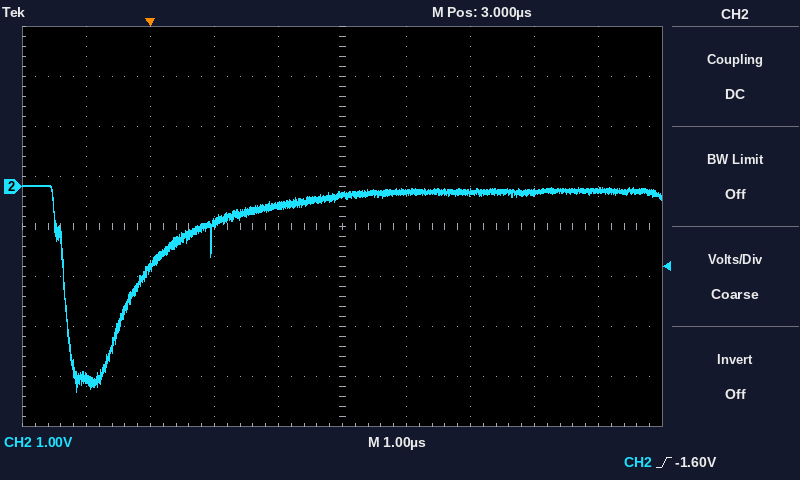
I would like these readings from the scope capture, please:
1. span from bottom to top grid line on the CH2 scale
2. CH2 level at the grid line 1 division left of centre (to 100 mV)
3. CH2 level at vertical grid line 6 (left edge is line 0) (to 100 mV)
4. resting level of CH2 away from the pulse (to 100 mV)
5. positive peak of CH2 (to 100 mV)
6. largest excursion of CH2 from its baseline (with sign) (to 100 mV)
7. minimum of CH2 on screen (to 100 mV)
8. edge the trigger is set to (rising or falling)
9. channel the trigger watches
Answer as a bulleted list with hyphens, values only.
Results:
- 8 V
- -400 mV
- -100 mV
- -100 mV
- 0.0 V
- -4.0 V
- -4.1 V
- rising
- CH2
